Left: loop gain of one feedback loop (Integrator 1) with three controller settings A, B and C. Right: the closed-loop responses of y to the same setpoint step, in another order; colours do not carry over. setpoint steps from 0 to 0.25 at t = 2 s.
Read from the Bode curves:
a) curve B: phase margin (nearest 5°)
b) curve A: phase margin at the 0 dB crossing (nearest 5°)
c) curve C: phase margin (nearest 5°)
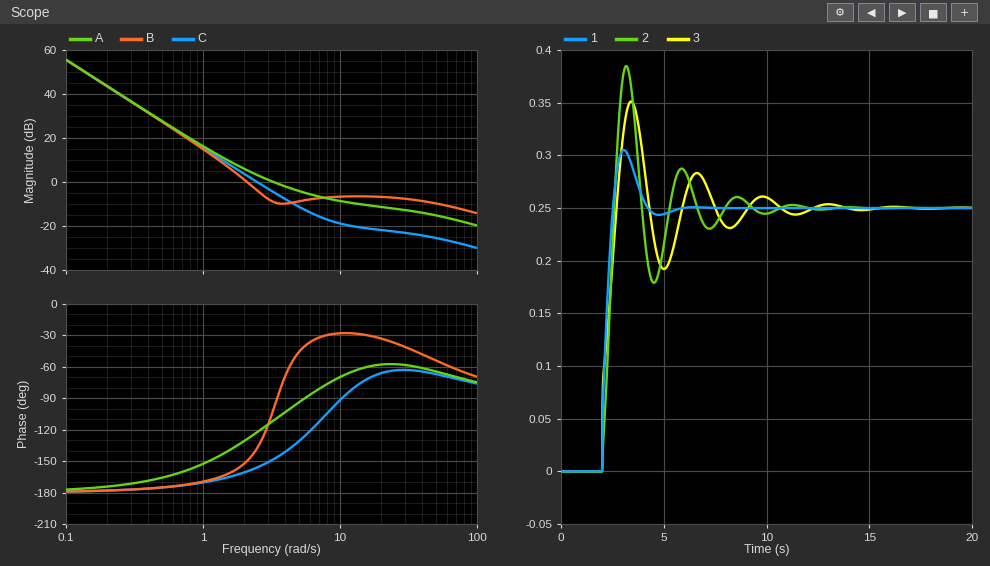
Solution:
30°
70°
25°
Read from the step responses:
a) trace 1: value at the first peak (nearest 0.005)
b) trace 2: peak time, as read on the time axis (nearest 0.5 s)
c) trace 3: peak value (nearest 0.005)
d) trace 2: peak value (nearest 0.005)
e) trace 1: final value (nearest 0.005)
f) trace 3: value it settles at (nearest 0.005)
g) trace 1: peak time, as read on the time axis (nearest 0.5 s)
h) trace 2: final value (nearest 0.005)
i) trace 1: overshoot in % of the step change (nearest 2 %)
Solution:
0.305
3.0 s
0.350
0.385
0.250
0.250
3.0 s
0.250
22 %
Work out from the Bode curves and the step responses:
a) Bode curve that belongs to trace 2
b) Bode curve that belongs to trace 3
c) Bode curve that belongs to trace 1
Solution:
C
B
A
